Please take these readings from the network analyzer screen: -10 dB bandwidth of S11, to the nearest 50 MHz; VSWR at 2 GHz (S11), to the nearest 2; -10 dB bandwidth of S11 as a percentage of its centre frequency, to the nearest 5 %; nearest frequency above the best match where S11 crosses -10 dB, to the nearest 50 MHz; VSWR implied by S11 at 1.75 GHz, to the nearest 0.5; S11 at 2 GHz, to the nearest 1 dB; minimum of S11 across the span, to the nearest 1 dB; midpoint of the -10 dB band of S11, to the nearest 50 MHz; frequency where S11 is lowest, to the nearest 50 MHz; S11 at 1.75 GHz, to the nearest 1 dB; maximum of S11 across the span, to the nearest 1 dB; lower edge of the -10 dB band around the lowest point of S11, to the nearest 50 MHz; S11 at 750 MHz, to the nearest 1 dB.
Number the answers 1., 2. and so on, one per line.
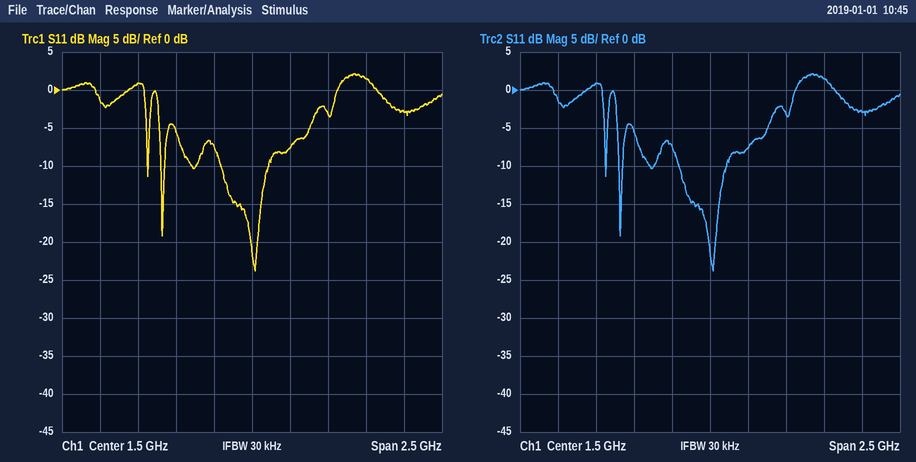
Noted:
1. 300 MHz
2. 6
3. 20 %
4. 1.60 GHz
5. 2.5
6. -3 dB
7. -24 dB
8. 1.45 GHz
9. 1.50 GHz
10. -8 dB
11. 2 dB
12. 1.30 GHz
13. 1 dB
